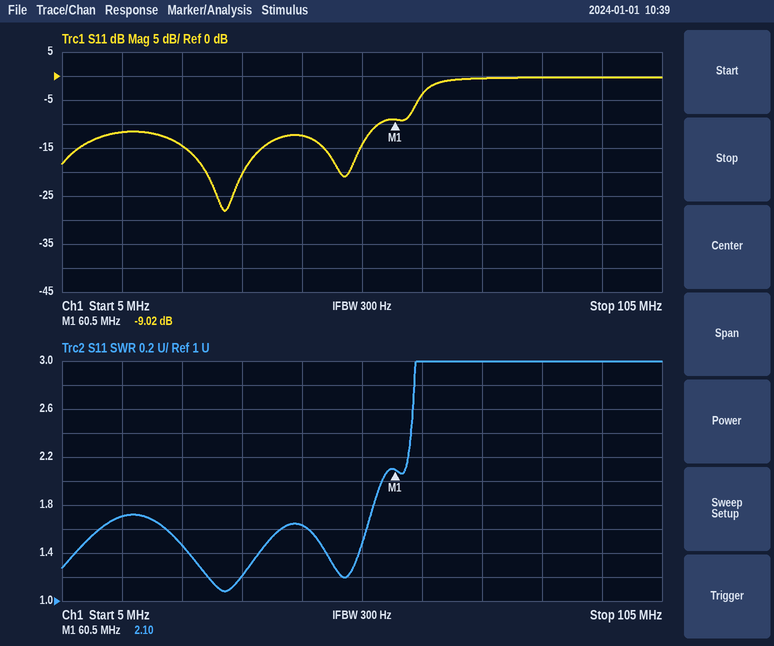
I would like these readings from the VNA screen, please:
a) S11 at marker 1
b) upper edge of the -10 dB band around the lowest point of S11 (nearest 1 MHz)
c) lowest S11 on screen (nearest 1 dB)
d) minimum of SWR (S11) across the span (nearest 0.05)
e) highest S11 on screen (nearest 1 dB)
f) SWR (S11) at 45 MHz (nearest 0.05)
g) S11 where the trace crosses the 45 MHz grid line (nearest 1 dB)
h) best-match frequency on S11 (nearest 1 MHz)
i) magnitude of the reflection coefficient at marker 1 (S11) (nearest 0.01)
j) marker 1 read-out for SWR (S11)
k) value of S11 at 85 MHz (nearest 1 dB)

-9.02 dB
58 MHz
-28 dB
1.10
0 dB
1.65
-12 dB
32 MHz
0.35
2.10
0 dB
